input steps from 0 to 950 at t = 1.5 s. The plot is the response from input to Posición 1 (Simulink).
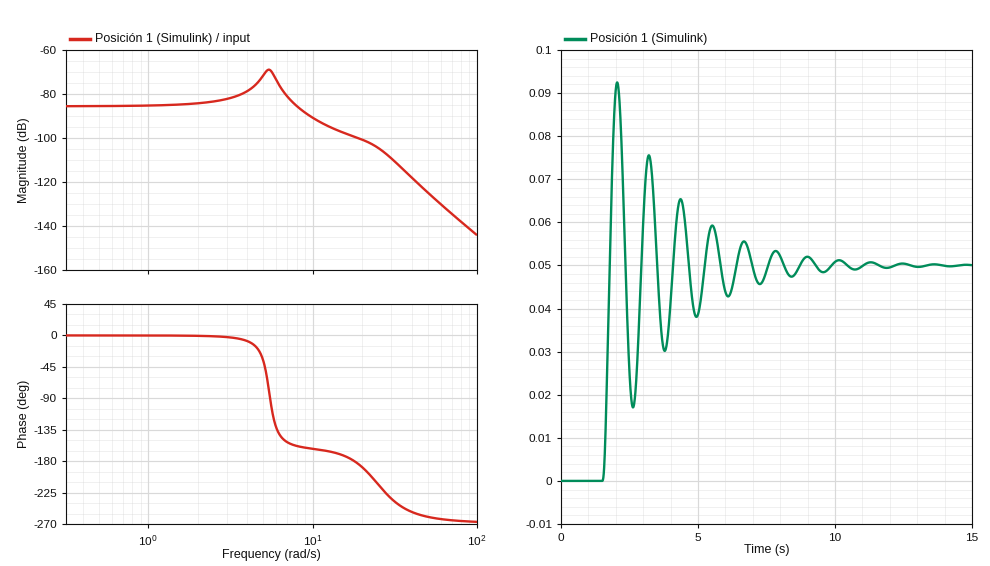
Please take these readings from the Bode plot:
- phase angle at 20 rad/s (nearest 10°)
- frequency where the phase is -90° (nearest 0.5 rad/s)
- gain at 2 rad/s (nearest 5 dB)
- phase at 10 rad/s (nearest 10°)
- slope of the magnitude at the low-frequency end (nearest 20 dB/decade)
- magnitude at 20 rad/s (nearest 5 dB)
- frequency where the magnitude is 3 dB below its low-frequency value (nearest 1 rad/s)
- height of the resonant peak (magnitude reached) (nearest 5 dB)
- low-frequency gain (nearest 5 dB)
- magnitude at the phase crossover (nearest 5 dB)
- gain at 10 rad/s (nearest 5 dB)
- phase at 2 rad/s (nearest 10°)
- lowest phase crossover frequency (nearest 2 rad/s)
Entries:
-190°
5.5 rad/s
-85 dB
-160°
0 dB/decade
-100 dB
9 rad/s
-70 dB
-85 dB
-100 dB
-90 dB
0°
18 rad/s
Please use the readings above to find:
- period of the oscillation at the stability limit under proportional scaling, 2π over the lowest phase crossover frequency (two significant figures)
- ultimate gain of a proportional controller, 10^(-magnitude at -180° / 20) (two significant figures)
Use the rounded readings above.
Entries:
0.35 s
100000
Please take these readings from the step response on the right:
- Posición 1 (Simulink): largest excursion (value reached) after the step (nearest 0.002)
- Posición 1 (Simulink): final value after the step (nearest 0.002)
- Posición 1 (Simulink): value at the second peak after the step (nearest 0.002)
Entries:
0.092
0.050
0.076
